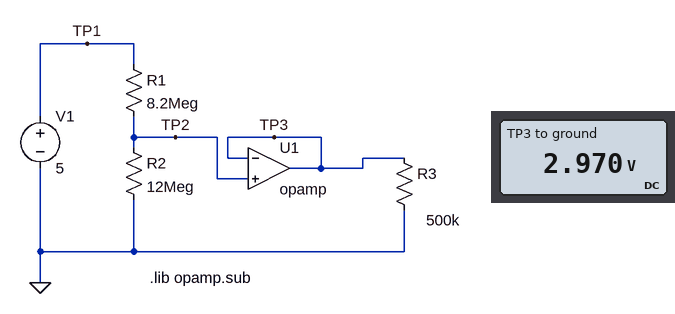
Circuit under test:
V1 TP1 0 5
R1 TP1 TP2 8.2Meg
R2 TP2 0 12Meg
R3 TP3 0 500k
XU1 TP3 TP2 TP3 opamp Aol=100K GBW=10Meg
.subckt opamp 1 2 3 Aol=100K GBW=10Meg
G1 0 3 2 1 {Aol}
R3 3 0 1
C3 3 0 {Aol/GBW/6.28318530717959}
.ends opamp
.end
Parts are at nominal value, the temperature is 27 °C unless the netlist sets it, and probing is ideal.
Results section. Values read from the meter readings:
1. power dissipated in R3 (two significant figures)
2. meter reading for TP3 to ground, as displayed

18 µW
2.970 V
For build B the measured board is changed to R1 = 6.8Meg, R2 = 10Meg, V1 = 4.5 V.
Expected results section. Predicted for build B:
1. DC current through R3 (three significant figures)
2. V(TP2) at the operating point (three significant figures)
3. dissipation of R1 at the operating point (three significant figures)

5.36 µA
2.68 V
488 nW
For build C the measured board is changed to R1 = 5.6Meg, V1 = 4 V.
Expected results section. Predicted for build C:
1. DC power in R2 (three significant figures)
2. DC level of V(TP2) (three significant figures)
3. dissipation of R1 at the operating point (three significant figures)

620 nW
2.73 V
289 nW
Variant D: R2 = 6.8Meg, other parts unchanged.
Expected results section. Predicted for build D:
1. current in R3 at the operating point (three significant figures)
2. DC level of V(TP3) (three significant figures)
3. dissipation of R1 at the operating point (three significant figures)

4.53 µA
2.27 V
911 nW
